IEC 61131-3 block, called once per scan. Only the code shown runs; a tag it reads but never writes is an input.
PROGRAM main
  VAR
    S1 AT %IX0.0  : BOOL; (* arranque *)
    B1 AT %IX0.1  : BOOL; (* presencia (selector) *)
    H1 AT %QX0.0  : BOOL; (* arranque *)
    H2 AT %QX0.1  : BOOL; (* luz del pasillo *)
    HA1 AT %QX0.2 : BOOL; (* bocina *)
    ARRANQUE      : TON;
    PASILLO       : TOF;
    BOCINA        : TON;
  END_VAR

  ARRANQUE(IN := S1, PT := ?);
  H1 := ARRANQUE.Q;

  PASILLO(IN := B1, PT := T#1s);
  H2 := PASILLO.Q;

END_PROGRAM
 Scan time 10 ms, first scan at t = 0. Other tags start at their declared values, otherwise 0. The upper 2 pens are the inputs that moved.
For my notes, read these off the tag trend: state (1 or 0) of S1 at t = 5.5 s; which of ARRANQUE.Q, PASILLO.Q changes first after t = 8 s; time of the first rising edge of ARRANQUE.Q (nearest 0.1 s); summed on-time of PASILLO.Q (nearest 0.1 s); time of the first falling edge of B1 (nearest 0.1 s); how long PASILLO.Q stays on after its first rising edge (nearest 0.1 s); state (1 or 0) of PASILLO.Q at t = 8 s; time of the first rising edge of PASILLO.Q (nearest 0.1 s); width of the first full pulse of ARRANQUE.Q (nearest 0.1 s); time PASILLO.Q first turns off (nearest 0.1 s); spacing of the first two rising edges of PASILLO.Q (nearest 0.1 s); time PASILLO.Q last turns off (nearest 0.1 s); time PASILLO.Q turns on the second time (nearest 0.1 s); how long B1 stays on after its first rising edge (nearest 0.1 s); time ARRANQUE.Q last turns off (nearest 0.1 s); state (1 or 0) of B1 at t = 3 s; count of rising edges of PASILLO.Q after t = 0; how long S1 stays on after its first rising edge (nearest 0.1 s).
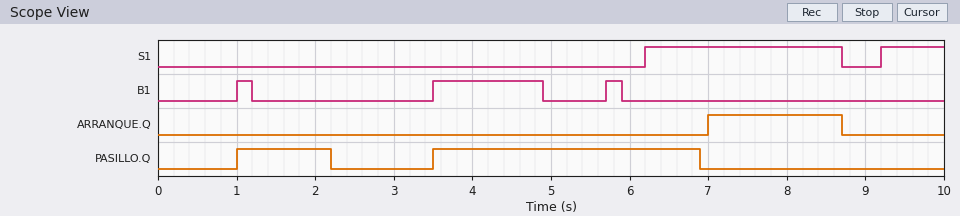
0
ARRANQUE.Q
7.0 s
4.6 s
1.2 s
1.2 s
0
1.0 s
1.7 s
2.2 s
2.5 s
6.9 s
3.5 s
0.2 s
8.7 s
0
2
2.5 s
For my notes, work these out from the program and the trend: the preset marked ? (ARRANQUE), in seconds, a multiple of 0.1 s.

0.8 s
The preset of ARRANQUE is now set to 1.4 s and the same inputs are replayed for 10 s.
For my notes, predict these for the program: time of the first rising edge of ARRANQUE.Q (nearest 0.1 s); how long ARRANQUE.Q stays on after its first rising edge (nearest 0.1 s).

7.6 s
1.1 s
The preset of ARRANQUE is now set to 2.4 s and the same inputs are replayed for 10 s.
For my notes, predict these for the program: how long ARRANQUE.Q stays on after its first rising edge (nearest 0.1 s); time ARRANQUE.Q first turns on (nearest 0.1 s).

0.1 s
8.6 s
